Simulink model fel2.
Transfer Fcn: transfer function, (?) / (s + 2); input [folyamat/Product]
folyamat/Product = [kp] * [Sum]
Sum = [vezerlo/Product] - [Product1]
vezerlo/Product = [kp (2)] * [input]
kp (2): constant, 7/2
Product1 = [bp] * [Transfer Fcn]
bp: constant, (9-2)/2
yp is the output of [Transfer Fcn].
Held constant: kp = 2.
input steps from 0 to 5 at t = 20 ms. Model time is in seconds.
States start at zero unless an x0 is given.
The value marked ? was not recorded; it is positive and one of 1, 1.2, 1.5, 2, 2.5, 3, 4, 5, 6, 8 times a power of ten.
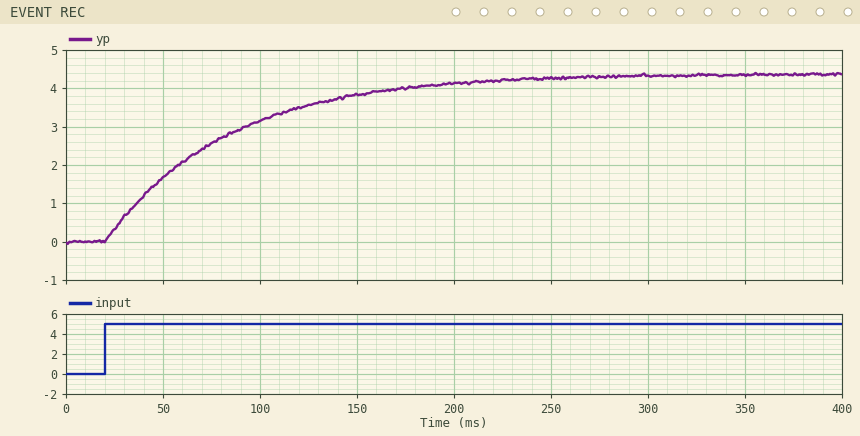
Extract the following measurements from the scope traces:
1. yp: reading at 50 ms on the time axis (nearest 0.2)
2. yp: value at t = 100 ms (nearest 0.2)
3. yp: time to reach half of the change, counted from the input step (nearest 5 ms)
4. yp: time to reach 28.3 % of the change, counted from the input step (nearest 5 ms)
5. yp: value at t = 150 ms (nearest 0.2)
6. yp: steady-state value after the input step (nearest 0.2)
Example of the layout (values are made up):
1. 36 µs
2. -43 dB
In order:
1. 1.6
2. 3.2
3. 45 ms
4. 20 ms
5. 3.8
6. 4.4
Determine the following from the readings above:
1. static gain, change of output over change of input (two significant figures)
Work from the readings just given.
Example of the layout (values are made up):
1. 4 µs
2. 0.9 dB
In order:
1. 0.88
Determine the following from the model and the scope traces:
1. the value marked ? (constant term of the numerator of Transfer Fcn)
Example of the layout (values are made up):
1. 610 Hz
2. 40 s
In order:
1. 2
